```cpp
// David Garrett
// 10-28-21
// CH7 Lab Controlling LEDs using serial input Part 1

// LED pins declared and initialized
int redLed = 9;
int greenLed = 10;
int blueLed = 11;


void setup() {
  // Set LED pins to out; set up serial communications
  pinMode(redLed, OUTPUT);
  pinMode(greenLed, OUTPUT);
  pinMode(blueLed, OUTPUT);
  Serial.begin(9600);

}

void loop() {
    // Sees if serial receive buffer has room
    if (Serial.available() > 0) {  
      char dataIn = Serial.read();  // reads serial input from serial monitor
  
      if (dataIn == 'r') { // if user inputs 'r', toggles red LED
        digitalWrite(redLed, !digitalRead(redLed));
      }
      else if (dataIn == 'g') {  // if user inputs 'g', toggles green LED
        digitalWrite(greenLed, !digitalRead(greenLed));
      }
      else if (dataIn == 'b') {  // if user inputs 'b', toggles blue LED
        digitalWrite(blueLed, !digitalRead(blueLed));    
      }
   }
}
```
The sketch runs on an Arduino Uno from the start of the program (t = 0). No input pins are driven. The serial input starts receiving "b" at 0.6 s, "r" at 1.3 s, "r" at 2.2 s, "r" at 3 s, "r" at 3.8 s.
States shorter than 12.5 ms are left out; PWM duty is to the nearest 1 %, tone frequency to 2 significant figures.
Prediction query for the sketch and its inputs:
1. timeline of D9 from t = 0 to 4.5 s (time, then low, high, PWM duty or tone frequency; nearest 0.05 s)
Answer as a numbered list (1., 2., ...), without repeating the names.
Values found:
1. 0 s low; 1.3 s high; 2.2 s low; 3 s high; 3.8 s low
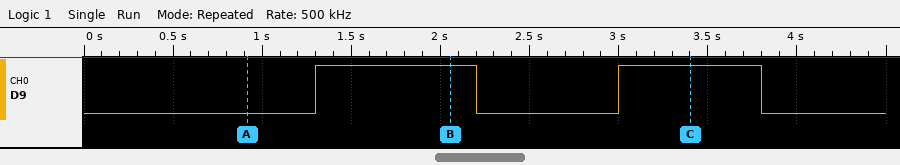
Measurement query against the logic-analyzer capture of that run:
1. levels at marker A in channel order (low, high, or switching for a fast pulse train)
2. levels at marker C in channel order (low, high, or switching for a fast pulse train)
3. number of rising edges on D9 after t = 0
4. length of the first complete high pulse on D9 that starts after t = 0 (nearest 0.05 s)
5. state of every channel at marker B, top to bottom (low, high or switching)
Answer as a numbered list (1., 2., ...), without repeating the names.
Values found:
1. D9 low
2. D9 high
3. 2
4. 0.90 s
5. D9 high
